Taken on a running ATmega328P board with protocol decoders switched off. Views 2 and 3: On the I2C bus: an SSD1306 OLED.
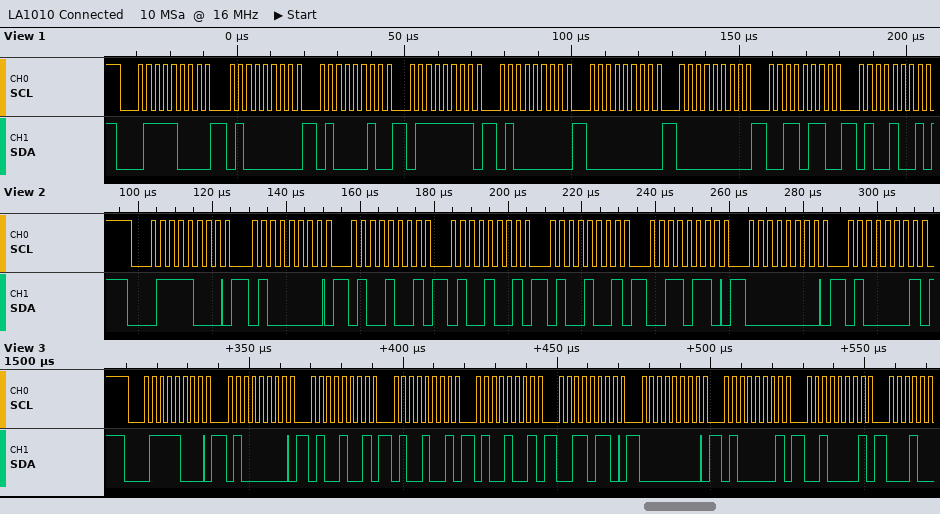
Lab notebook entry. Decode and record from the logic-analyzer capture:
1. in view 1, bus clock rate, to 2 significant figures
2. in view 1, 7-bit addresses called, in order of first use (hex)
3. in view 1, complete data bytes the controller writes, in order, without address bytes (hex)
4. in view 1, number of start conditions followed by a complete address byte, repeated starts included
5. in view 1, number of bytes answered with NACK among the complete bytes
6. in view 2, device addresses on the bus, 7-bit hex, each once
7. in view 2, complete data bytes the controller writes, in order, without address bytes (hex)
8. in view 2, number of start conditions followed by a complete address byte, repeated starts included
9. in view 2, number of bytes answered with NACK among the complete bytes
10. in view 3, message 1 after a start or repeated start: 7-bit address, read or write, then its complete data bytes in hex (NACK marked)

400 kHz
0x3C
40 42 7F 40 00 00 36 49
1
0
0x3C
40 49 49 49 36 00 41
1
0
0x3C write: 40 49 49 49 36 00 41 21
